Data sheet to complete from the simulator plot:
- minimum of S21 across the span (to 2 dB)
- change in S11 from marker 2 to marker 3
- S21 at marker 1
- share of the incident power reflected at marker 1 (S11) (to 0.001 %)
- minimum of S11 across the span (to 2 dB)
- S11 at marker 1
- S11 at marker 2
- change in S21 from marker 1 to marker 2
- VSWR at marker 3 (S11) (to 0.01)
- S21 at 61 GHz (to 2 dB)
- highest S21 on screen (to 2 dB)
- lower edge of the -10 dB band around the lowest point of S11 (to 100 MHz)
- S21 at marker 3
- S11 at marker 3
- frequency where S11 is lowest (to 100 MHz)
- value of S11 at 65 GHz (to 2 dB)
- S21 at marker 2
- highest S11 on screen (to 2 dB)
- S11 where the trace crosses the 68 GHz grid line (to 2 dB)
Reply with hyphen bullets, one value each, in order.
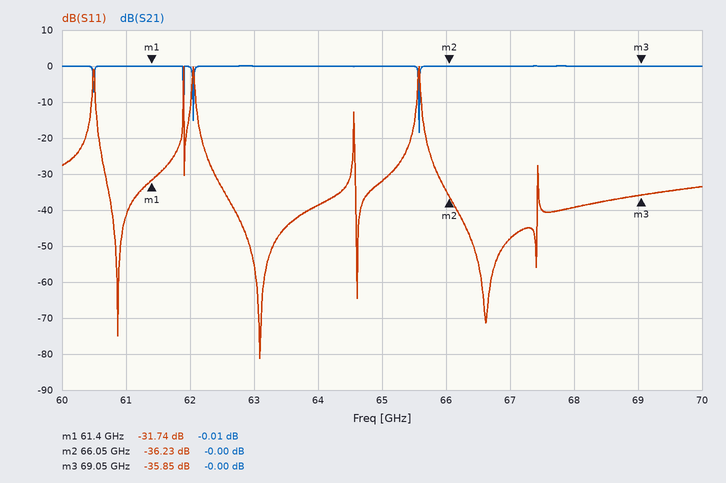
- -18 dB
- 0.38 dB
- -0.01 dB
- 0.067 %
- -82 dB
- -31.74 dB
- -36.23 dB
- 0.01 dB
- 1.03
- 0 dB
- 0 dB
- 62.1 GHz
- -0.00 dB
- -35.85 dB
- 63.1 GHz
- -32 dB
- -0.00 dB
- 0 dB
- -40 dB
